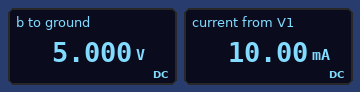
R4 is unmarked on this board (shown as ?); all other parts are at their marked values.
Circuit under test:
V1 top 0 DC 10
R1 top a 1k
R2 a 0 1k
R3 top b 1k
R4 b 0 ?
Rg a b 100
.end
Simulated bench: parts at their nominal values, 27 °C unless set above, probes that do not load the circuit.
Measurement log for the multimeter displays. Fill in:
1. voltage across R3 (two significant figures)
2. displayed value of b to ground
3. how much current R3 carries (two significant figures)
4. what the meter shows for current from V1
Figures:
5.0 V
5.000 V
5.0 mA
10.00 mA
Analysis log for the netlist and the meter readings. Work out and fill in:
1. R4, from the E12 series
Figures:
1 kΩ
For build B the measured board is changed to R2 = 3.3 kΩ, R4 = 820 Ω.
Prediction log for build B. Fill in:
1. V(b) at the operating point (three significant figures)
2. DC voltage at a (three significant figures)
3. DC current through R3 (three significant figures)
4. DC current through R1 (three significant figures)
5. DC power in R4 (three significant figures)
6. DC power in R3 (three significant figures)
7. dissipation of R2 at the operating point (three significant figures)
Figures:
5.59 V
5.83 V
4.41 mA
4.17 mA
38.1 mW
19.5 mW
10.3 mW
